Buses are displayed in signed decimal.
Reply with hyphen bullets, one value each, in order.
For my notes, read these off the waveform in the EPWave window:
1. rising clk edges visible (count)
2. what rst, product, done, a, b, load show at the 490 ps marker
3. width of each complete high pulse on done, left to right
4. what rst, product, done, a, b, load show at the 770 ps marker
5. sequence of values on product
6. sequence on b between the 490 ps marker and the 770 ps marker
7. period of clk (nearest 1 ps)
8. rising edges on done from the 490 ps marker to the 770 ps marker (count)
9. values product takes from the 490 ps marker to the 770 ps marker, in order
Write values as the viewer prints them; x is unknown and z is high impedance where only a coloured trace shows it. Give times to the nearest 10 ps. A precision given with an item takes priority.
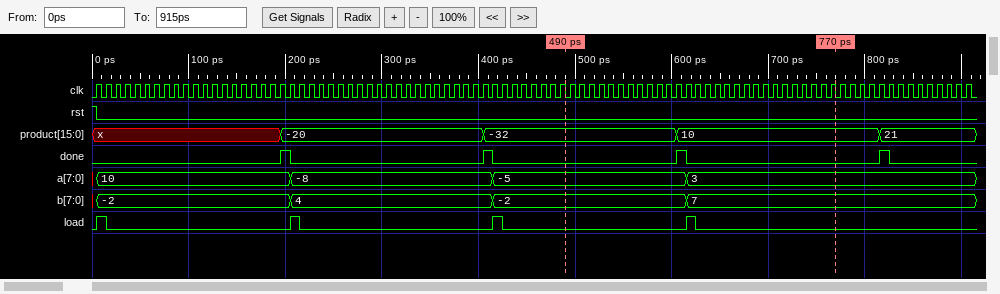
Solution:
- 91
- rst=0, product=-32, done=0, a=-5, b=-2, load=0
- 10 ps, 10 ps, 10 ps, 10 ps
- rst=0, product=10, done=0, a=3, b=7, load=0
- x, -20, -32, 10, 21
- -2, 7
- 10 ps
- 1
- -32, 10
